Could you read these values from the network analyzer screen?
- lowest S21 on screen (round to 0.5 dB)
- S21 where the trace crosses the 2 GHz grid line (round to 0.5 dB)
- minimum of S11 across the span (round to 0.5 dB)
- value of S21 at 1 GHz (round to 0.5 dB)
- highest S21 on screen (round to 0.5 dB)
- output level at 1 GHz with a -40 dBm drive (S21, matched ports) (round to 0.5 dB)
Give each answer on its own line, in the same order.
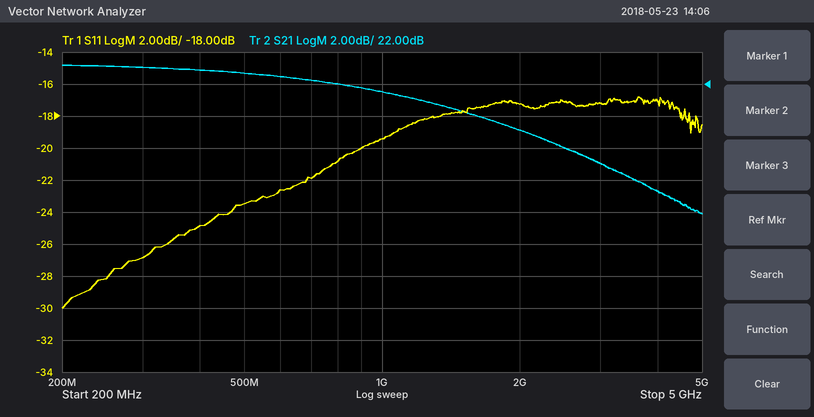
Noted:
14.0 dB
19.0 dB
-30.0 dB
21.5 dB
23.0 dB
-18.5 dBm
